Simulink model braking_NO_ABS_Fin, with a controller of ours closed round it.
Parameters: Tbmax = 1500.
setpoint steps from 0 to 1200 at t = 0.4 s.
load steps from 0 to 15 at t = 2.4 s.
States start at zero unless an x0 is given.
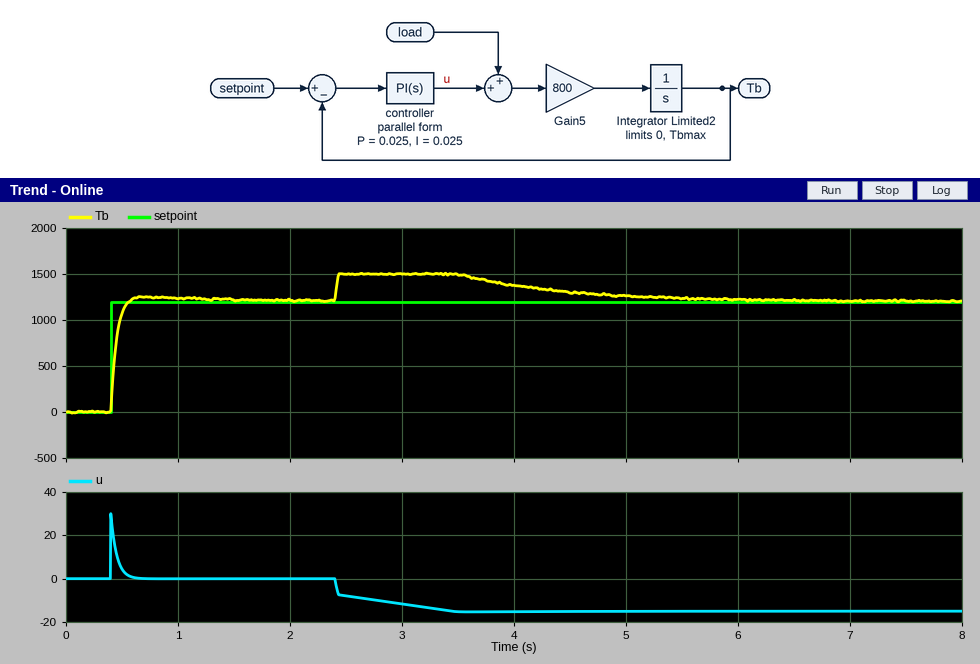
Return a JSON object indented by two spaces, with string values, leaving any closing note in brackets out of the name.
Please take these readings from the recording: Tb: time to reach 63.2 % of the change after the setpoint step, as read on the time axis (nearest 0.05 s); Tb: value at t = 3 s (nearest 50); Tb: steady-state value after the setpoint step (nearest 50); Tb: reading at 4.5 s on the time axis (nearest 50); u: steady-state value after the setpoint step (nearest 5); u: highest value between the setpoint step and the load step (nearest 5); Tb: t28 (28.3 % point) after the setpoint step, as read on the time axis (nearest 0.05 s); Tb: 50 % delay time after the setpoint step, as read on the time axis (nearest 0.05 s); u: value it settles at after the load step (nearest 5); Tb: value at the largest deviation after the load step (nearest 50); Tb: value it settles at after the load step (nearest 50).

{
  "Tb: time to reach 63.2 % of the change after the setpoint step, as read on the time axis": "0.45 s",
  "Tb: value at t = 3 s": "1500",
  "Tb: steady-state value after the setpoint step": "1200",
  "Tb: reading at 4.5 s on the time axis": "1300",
  "u: steady-state value after the setpoint step": "0",
  "u: highest value between the setpoint step and the load step": "30",
  "Tb: t28 (28.3 % point) after the setpoint step, as read on the time axis": "0.40 s",
  "Tb: 50 % delay time after the setpoint step, as read on the time axis": "0.45 s",
  "u: value it settles at after the load step": "-15",
  "Tb: value at the largest deviation after the load step": "1500",
  "Tb: value it settles at after the load step": "1200"
}
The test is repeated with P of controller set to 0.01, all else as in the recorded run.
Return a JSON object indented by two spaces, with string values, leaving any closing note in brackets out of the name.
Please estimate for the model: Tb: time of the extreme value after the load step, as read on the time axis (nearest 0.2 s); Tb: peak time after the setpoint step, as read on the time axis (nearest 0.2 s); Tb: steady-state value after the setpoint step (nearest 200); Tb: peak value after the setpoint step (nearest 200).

{
  "Tb: time of the extreme value after the load step, as read on the time axis": "2.4 s",
  "Tb: peak time after the setpoint step, as read on the time axis": "0.8 s",
  "Tb: steady-state value after the setpoint step": "1200",
  "Tb: peak value after the setpoint step": "1400"
}
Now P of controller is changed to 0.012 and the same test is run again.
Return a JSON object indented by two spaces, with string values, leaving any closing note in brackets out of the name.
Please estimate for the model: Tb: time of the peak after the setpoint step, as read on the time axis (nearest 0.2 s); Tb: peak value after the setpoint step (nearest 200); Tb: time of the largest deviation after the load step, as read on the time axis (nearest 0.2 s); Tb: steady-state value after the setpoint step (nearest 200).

{
  "Tb: time of the peak after the setpoint step, as read on the time axis": "0.8 s",
  "Tb: peak value after the setpoint step": "1400",
  "Tb: time of the largest deviation after the load step, as read on the time axis": "2.4 s",
  "Tb: steady-state value after the setpoint step": "1200"
}
